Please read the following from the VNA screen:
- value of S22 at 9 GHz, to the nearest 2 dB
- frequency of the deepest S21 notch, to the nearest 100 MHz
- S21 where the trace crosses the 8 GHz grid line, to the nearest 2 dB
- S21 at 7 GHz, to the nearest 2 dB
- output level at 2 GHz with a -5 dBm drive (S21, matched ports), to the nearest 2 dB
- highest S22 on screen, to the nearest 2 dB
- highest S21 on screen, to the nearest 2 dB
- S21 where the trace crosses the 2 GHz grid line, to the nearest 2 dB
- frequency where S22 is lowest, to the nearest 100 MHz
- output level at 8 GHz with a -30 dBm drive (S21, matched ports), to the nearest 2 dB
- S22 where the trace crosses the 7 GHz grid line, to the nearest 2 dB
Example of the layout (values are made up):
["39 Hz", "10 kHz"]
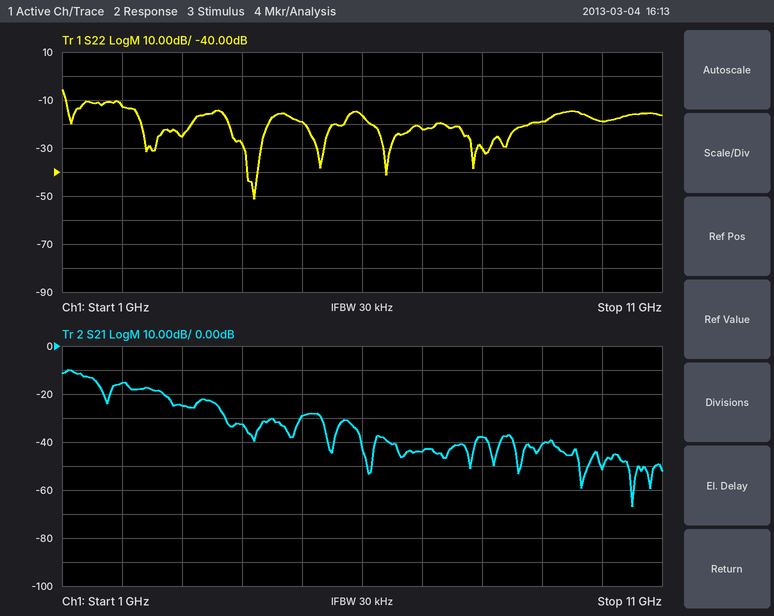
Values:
["-18 dB", "10.5 GHz", "-38 dB", "-44 dB", "-20 dBm", "-6 dB", "-10 dB", "-16 dB", "4.2 GHz", "-68 dBm", "-22 dB"]
